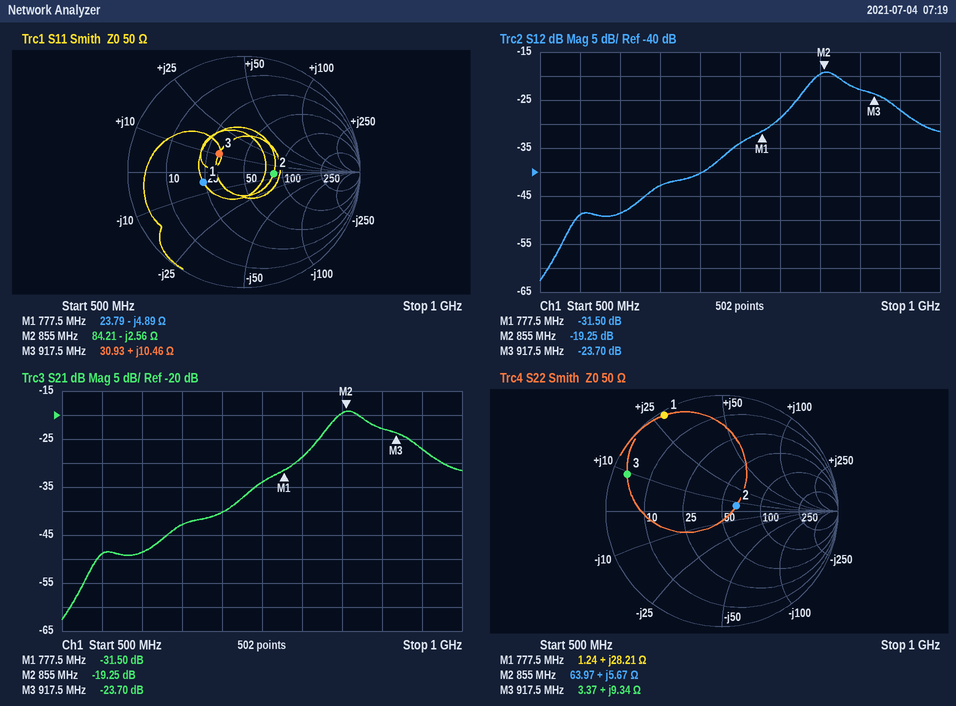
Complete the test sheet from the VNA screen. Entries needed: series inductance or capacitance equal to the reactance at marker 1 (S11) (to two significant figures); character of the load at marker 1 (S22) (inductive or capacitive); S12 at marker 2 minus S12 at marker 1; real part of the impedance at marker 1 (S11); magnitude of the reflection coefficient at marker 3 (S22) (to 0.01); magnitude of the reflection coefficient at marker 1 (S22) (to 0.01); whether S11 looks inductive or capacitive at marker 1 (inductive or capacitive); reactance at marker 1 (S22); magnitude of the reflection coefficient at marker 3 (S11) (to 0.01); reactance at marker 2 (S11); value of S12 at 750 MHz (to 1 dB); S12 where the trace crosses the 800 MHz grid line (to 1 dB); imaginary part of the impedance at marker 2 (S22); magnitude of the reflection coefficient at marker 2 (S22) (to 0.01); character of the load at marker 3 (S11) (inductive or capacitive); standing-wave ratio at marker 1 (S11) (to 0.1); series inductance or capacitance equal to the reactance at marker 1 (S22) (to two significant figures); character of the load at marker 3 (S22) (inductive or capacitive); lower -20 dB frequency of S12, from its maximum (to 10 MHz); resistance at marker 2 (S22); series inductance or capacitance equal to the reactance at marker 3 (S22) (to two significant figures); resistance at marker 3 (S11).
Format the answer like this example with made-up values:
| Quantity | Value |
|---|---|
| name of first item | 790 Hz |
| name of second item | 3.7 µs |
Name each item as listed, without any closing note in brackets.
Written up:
| Quantity | Value |
|---|---|
| series inductance or capacitance equal to the reactance at marker 1 (S11) | 42 pF |
| character of the load at marker 1 (S22) | inductive |
| S12 at marker 2 minus S12 at marker 1 | 12.25 dB |
| real part of the impedance at marker 1 | 23.79 Ω |
| magnitude of the reflection coefficient at marker 3 (S22) | 0.88 |
| magnitude of the reflection coefficient at marker 1 (S22) | 0.96 |
| whether S11 looks inductive or capacitive at marker 1 | capacitive |
| reactance at marker 1 | +28.21 Ω |
| magnitude of the reflection coefficient at marker 3 (S11) | 0.27 |
| reactance at marker 2 | -2.56 Ω |
| value of S12 at 750 MHz | -34 dB |
| S12 where the trace crosses the 800 MHz grid line | -29 dB |
| imaginary part of the impedance at marker 2 | +5.67 Ω |
| magnitude of the reflection coefficient at marker 2 (S22) | 0.13 |
| character of the load at marker 3 (S11) | inductive |
| standing-wave ratio at marker 1 (S11) | 2.1 |
| series inductance or capacitance equal to the reactance at marker 1 (S22) | 5.8 nH |
| character of the load at marker 3 (S22) | inductive |
| lower -20 dB frequency of S12, from its maximum | 710 MHz |
| resistance at marker 2 | 63.97 Ω |
| series inductance or capacitance equal to the reactance at marker 3 (S22) | 1.6 nH |
| resistance at marker 3 | 30.93 Ω |
